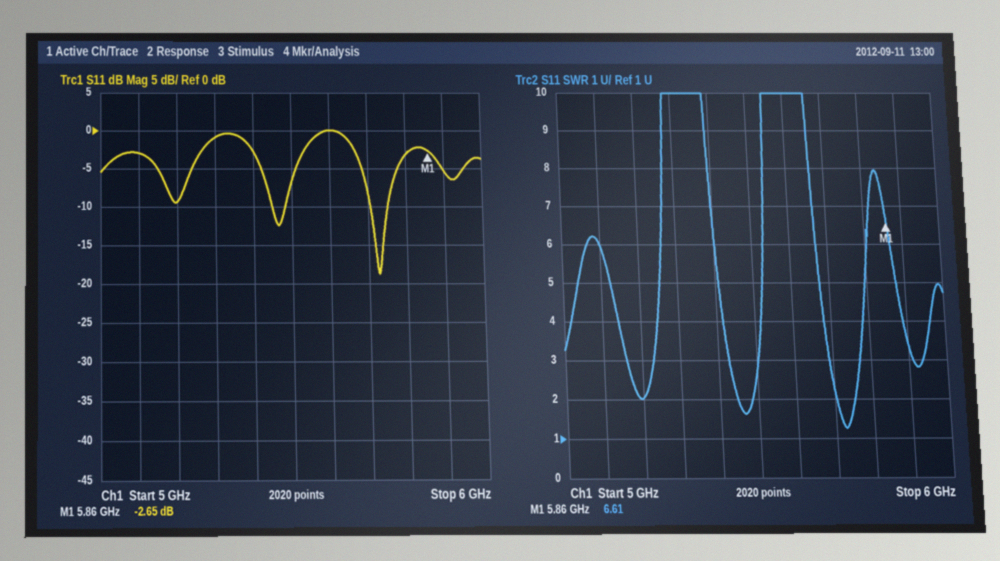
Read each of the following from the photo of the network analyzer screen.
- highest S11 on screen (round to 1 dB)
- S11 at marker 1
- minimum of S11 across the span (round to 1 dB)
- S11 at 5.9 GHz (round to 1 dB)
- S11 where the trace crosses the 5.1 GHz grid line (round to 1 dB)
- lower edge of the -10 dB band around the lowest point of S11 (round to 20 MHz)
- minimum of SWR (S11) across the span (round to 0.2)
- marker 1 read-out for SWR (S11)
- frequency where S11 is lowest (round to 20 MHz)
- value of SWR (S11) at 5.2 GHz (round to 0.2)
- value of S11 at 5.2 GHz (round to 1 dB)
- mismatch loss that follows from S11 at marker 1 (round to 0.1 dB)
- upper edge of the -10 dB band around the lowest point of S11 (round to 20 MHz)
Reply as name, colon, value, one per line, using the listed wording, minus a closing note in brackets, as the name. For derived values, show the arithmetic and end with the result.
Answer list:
highest S11 on screen: 0 dB
S11 at marker 1: -2.65 dB
minimum of S11 across the span: -19 dB
S11 at 5.9 GHz: -5 dB
S11 where the trace crosses the 5.1 GHz grid line: -3 dB
lower edge of the -10 dB band around the lowest point of S11: 5.70 GHz
minimum of SWR (S11) across the span: 1.2
marker 1 read-out for SWR: 6.61
frequency where S11 is lowest: 5.72 GHz
value of SWR (S11) at 5.2 GHz: 2.0
value of S11 at 5.2 GHz: -9 dB
mismatch loss that follows from S11 at marker 1: −10 log10(1 − 10^(-2.65/10)) ≈ 3.4 dB
upper edge of the -10 dB band around the lowest point of S11: 5.76 GHz
